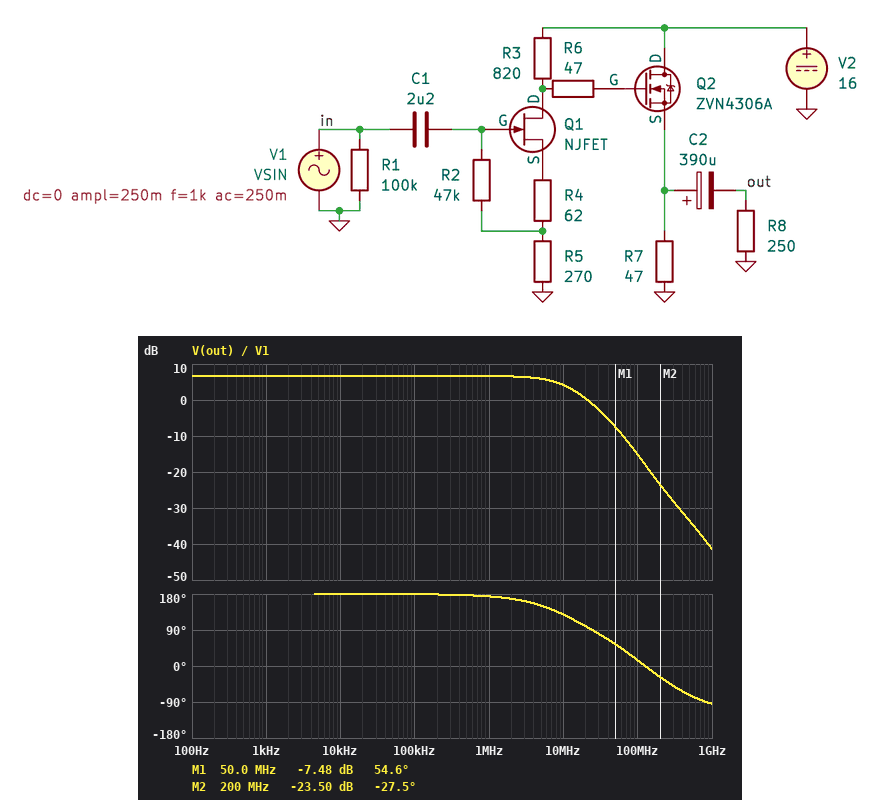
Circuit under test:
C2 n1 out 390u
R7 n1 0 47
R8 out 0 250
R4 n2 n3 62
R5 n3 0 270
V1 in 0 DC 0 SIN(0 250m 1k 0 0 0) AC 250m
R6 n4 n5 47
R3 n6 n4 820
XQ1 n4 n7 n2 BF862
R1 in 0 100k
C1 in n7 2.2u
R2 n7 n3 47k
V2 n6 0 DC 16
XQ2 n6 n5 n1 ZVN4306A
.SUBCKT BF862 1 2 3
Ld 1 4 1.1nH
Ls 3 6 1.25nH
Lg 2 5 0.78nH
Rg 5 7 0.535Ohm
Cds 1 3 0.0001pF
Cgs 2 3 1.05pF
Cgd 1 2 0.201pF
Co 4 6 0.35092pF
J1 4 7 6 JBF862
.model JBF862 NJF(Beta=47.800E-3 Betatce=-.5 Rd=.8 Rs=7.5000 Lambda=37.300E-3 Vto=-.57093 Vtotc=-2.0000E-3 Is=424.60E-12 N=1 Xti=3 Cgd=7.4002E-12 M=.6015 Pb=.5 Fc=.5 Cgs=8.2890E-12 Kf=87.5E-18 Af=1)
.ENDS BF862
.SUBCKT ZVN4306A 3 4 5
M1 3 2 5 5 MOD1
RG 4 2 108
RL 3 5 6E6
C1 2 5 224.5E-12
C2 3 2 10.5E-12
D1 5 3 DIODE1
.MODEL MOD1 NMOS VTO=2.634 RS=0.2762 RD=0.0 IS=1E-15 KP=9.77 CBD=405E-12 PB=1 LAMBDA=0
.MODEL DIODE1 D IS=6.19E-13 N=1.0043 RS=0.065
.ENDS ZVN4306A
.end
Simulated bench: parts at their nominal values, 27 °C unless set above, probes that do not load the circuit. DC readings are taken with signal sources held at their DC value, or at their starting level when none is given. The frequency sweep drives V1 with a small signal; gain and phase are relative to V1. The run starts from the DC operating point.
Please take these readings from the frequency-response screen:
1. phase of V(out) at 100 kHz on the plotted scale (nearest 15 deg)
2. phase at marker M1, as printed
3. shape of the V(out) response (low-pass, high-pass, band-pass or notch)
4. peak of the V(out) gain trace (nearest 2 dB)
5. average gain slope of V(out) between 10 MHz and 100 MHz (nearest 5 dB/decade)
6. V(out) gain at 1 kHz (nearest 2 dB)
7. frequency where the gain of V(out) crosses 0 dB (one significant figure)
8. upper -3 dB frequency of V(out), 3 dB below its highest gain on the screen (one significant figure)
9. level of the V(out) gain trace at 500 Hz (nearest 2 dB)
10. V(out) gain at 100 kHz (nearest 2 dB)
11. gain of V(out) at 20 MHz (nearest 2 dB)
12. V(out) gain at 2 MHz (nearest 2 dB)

180 deg
54.6 deg
low-pass
6 dB
-20 dB/decade
6 dB
20 MHz
10 MHz
6 dB
6 dB
0 dB
6 dB
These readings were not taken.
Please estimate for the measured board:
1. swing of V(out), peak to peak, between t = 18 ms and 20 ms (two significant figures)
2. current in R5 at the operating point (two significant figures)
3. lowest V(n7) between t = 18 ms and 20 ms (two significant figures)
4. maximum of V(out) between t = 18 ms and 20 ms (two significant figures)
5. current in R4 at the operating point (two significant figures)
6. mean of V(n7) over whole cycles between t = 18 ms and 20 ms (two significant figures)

1.1 V
4.5 mA
960 mV
540 mV
4.5 mA
1.2 V
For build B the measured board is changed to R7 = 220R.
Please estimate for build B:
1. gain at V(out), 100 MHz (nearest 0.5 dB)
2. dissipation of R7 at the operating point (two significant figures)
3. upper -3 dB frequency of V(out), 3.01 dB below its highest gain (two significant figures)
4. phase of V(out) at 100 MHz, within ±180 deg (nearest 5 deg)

-18.5 dB
420 mW
14 MHz
0 deg
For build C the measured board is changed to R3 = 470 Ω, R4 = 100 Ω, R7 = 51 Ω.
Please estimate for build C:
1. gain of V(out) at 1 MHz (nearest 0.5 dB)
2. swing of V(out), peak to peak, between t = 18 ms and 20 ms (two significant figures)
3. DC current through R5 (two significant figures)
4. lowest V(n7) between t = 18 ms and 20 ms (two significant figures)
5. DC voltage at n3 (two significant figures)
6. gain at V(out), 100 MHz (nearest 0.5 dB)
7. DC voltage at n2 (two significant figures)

1.0 dB
560 mV
3.3 mA
640 mV
890 mV
-17.0 dB
1.2 V
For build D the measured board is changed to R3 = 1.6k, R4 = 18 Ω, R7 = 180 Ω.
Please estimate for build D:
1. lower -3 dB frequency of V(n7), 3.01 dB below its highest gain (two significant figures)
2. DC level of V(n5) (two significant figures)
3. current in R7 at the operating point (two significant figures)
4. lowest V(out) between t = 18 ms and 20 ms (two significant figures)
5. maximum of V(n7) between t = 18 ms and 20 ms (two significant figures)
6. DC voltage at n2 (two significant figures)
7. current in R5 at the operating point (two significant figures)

290 mHz
4.1 V
7.9 mA
-830 mV
2.3 V
2.1 V
7.4 mA
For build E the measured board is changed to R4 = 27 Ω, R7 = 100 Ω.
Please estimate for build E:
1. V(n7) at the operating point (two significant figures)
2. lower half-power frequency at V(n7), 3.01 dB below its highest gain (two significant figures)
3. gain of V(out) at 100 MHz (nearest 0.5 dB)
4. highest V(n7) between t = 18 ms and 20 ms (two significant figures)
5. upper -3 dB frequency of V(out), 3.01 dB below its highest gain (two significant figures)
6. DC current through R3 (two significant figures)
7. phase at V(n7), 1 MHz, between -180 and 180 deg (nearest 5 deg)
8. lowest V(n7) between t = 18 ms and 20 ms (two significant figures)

1.9 V
290 mHz
-15.5 dB
2.1 V
12 MHz
6.9 mA
0 deg
1.6 V
